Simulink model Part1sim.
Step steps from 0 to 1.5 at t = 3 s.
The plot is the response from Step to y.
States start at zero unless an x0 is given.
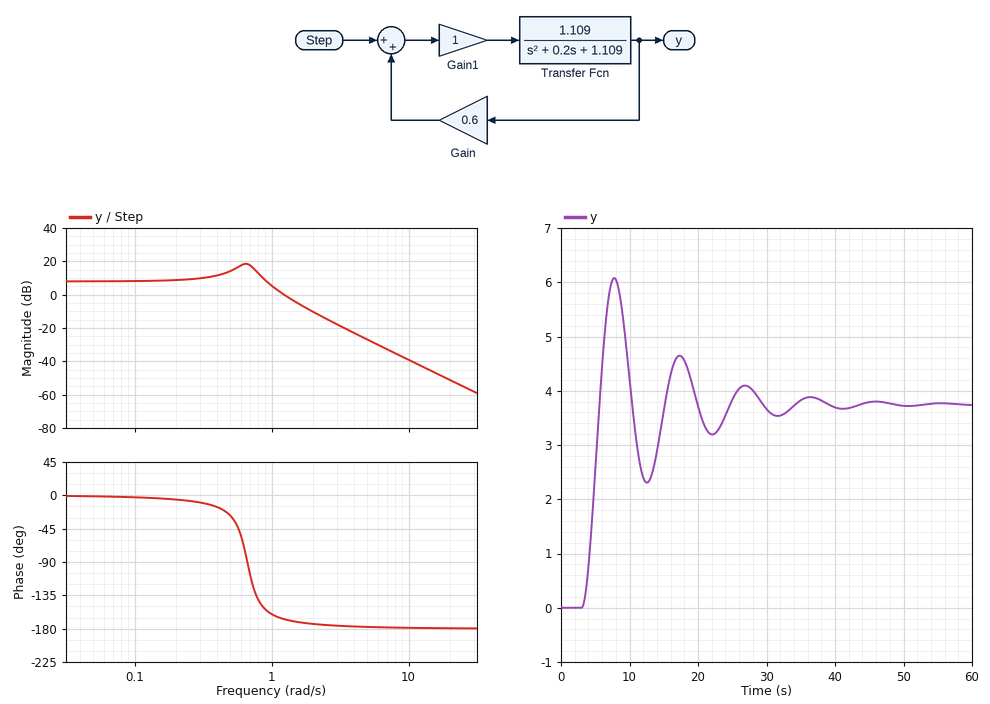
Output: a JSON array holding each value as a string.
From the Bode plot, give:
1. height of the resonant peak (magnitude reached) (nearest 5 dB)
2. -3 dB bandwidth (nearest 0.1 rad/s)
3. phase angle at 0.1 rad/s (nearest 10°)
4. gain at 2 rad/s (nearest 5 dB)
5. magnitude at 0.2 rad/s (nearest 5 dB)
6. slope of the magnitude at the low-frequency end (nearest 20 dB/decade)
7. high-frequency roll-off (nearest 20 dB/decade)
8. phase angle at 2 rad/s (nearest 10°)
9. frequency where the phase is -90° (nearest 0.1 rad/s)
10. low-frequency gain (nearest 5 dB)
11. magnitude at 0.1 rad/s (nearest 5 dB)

["20 dB", "1.0 rad/s", "0°", "-10 dB", "10 dB", "0 dB/decade", "-40 dB/decade", "-170°", "0.7 rad/s", "10 dB", "10 dB"]
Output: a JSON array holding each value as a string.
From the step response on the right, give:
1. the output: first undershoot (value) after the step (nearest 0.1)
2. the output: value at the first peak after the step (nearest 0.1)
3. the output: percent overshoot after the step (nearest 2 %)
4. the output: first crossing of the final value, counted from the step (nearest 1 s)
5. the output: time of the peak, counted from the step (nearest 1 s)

["2.3", "6.1", "62 %", "3 s", "5 s"]
